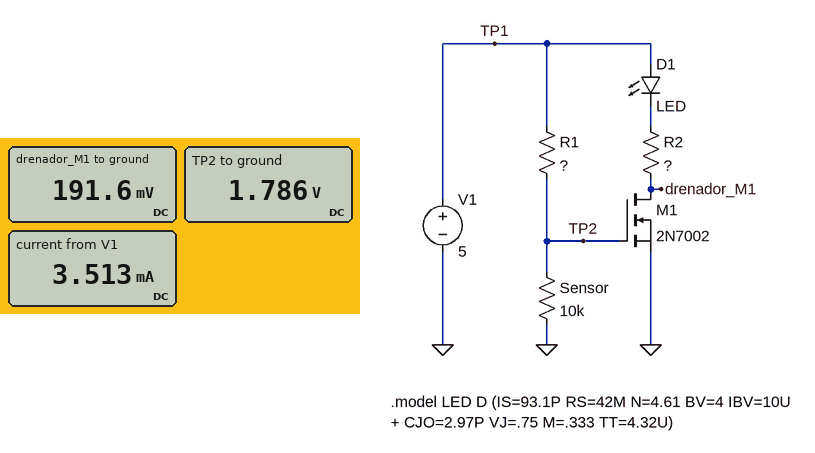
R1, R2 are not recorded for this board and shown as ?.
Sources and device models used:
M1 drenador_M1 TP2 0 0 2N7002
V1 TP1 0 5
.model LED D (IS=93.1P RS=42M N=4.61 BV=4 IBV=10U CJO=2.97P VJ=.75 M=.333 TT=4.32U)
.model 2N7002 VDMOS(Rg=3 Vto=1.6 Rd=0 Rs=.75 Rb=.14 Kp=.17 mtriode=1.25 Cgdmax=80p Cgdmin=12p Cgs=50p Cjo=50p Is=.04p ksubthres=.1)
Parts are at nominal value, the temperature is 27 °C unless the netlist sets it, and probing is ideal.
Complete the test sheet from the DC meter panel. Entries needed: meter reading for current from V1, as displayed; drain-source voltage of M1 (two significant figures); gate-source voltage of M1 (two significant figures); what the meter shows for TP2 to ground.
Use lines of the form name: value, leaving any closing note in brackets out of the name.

meter reading for current from V1, as displayed: 3.513 mA
drain-source voltage of M1: 190 mV
gate-source voltage of M1: 1.8 V
what the meter shows for TP2 to ground: 1.786 V
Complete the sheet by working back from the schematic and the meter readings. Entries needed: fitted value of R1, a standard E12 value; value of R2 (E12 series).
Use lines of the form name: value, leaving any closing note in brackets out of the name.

fitted value of R1, a standard E12 value: 18 kΩ
value of R2: 820 Ω
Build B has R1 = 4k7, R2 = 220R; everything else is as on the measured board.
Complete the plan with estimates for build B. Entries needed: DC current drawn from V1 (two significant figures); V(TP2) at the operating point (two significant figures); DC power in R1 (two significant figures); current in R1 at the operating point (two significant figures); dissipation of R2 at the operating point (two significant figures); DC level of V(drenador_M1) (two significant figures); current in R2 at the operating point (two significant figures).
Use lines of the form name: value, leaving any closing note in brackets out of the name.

DC current drawn from V1: 13 mA
V(TP2) at the operating point: 3.4 V
DC power in R1: 540 µW
current in R1 at the operating point: 340 µA
dissipation of R2 at the operating point: 34 mW
DC level of V(drenador_M1): 42 mV
current in R2 at the operating point: 12 mA
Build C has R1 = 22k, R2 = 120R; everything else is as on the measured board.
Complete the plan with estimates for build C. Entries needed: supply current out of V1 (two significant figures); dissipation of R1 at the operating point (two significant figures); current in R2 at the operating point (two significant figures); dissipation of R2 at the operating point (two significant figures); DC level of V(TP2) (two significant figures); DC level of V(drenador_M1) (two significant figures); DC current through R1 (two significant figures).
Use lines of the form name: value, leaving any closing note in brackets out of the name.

supply current out of V1: 390 µA
dissipation of R1 at the operating point: 540 µW
current in R2 at the operating point: 230 µA
dissipation of R2 at the operating point: 6.5 µW
DC level of V(TP2): 1.6 V
DC level of V(drenador_M1): 3.2 V
DC current through R1: 160 µA
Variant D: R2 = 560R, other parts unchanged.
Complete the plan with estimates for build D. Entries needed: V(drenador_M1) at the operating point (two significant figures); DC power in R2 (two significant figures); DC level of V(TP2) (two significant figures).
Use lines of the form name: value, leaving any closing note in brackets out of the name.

V(drenador_M1) at the operating point: 1.1 V
DC power in R2: 6.2 mW
DC level of V(TP2): 1.8 V
